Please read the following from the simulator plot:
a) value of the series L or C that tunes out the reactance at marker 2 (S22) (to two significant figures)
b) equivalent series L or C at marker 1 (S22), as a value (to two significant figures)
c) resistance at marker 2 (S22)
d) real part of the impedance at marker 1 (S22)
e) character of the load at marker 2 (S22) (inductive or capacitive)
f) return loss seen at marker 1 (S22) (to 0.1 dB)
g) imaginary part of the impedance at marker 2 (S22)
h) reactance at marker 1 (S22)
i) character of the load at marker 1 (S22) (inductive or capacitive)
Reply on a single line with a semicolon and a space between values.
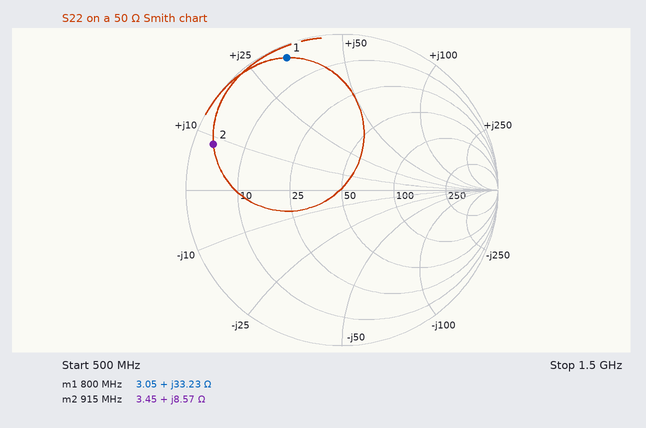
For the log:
20 pF; 6.6 nH; 3.45 Ω; 3.05 Ω; inductive; 0.7 dB; +8.57 Ω; +33.23 Ω; inductive
